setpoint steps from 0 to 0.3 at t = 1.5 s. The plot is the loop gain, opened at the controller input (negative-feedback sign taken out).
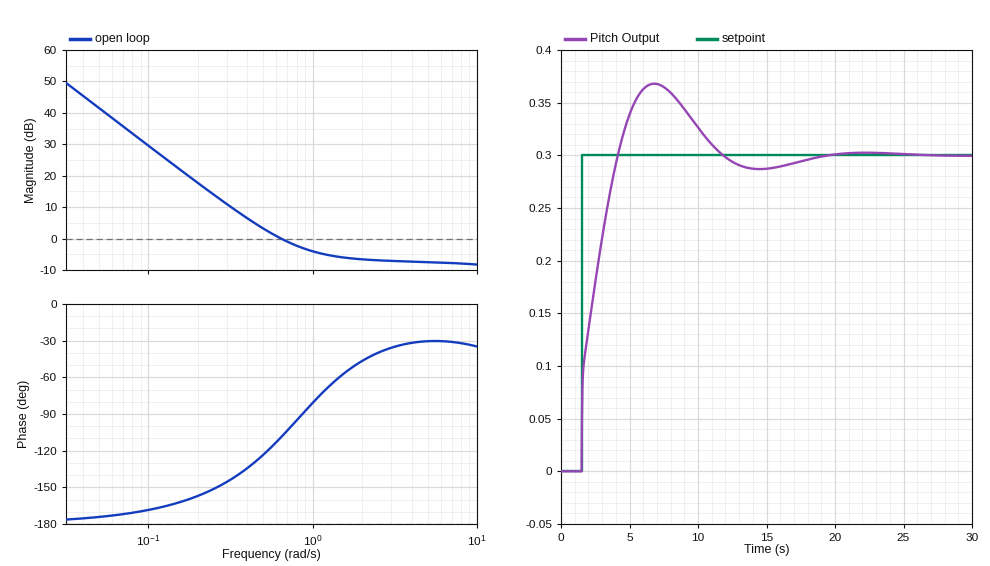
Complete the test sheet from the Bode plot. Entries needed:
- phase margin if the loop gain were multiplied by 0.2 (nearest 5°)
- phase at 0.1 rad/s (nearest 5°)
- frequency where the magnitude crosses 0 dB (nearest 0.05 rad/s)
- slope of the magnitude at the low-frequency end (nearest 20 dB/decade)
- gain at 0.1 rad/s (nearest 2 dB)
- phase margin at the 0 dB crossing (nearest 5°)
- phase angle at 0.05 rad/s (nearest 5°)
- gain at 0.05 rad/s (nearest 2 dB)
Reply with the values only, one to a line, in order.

30°
-170°
0.65 rad/s
-40 dB/decade
30 dB
70°
-175°
42 dB
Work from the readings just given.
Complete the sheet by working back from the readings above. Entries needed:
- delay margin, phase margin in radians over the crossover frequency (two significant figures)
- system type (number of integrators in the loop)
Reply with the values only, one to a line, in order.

1.9 s
2
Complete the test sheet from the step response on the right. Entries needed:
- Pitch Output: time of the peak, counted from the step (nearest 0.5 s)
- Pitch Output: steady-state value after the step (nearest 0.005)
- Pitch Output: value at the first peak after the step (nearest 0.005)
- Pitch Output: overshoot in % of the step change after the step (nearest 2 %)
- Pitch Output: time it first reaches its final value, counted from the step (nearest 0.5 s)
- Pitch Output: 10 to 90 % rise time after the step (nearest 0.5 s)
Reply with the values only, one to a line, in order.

5.5 s
0.300
0.370
22 %
2.5 s
2.0 s
